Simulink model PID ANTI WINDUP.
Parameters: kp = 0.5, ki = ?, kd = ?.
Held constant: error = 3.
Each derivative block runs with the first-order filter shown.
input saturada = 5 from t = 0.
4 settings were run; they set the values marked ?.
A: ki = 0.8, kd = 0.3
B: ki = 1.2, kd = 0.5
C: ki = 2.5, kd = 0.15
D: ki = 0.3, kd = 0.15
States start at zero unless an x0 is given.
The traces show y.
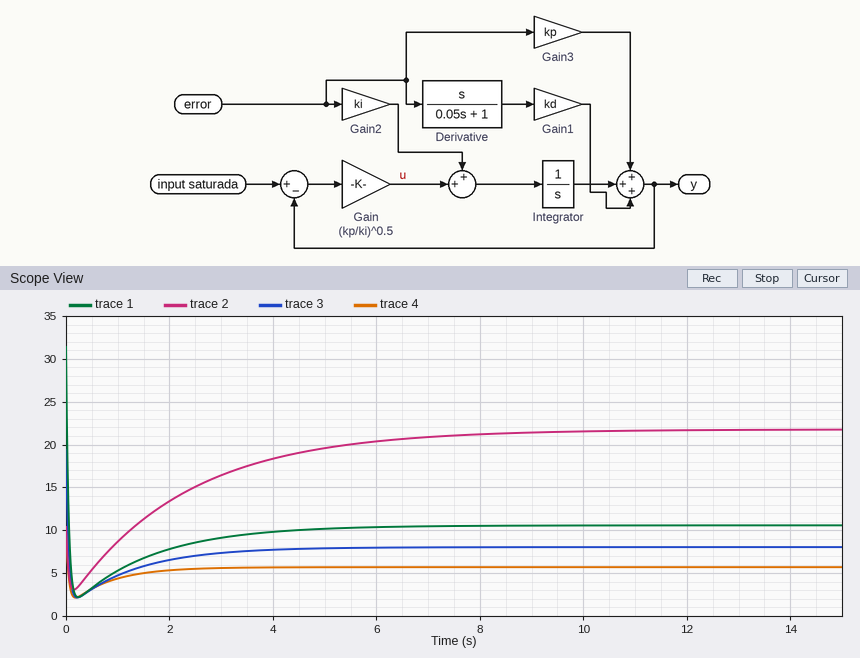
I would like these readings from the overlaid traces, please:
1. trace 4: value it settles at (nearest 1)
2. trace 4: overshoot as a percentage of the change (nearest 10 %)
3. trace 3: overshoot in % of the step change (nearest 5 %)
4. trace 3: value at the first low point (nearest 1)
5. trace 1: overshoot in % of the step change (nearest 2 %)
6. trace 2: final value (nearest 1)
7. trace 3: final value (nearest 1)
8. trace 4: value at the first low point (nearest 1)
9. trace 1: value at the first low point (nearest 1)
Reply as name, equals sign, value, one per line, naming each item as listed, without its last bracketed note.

trace 4: value it settles at = 6
trace 4: overshoot as a percentage of the change = 70 %
trace 3: overshoot in % of the step change = 50 %
trace 3: value at the first low point = 2
trace 1: overshoot in % of the step change = 40 %
trace 2: final value = 22
trace 3: final value = 8
trace 4: value at the first low point = 2
trace 1: value at the first low point = 2
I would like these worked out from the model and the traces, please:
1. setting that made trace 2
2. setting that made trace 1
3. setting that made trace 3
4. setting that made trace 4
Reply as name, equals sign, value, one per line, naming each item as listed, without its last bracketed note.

setting that made trace 2 = C
setting that made trace 1 = B
setting that made trace 3 = A
setting that made trace 4 = D
